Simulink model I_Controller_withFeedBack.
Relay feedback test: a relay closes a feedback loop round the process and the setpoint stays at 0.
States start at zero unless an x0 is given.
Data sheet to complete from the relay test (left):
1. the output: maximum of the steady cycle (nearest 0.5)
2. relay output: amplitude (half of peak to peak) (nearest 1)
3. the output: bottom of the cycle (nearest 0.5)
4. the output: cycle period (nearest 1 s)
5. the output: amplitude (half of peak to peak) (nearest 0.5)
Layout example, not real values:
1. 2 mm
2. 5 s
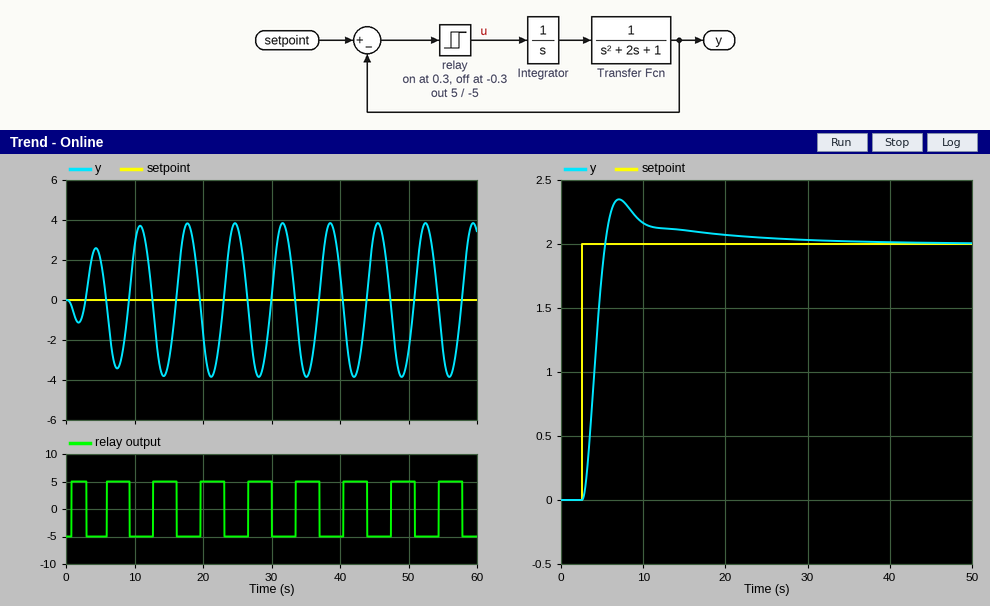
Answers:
1. 4.0
2. 5
3. -4.0
4. 7 s
5. 4.0
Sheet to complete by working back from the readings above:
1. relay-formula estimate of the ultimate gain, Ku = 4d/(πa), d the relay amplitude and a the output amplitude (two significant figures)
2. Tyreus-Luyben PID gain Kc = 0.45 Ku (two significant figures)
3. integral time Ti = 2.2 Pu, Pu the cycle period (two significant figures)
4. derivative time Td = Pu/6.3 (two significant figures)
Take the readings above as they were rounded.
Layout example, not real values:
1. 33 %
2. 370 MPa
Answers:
1. 1.6
2. 0.72
3. 15 s
4. 1.1 s
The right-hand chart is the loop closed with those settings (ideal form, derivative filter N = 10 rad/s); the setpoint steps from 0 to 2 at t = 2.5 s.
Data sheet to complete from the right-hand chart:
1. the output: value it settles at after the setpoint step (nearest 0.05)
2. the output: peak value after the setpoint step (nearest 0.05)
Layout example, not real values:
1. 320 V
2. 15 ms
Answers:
1. 2.00
2. 2.35
